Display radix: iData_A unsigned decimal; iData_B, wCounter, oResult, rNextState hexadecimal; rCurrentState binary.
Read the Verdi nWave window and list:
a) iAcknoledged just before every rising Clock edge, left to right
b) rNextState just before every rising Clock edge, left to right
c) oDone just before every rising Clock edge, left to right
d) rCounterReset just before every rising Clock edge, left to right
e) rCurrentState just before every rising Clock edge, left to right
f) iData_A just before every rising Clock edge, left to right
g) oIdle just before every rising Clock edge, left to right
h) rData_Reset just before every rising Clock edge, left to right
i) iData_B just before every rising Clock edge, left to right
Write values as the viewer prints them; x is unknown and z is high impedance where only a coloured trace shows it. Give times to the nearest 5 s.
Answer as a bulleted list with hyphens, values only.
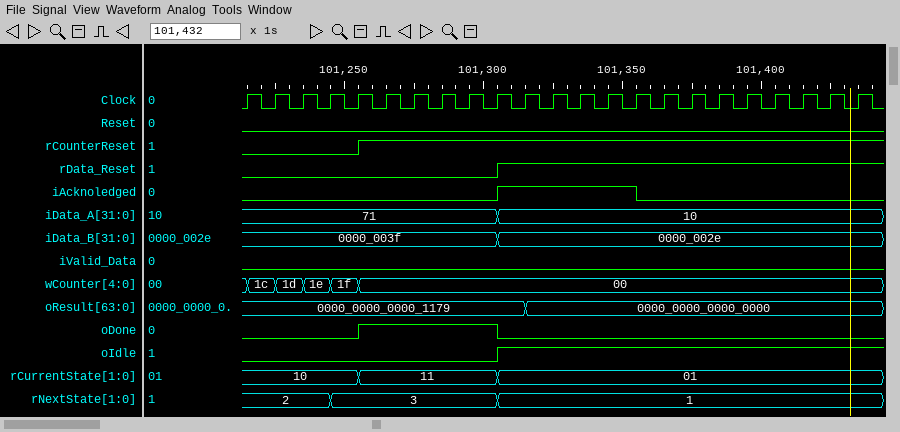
- 0 0 0 0 0 0 0 0 0 0 1 1 1 1 1 0 0 0 0 0 0 0 0
- 2, 2, 2, 2, 3, 3, 3, 3, 3, 3, 1, 1, 1, 1, 1, 1, 1, 1, 1, 1, 1, 1, 1
- 0 0 0 0 0 1 1 1 1 1 0 0 0 0 0 0 0 0 0 0 0 0 0
- 0 0 0 0 0 1 1 1 1 1 1 1 1 1 1 1 1 1 1 1 1 1 1
- 10, 10, 10, 10, 10, 11, 11, 11, 11, 11, 01, 01, 01, 01, 01, 01, 01, 01, 01, 01, 01, 01, 01
- 71, 71, 71, 71, 71, 71, 71, 71, 71, 71, 10, 10, 10, 10, 10, 10, 10, 10, 10, 10, 10, 10, 10
- 0 0 0 0 0 0 0 0 0 0 1 1 1 1 1 1 1 1 1 1 1 1 1
- 0 0 0 0 0 0 0 0 0 0 1 1 1 1 1 1 1 1 1 1 1 1 1
- 0000_003f, 0000_003f, 0000_003f, 0000_003f, 0000_003f, 0000_003f, 0000_003f, 0000_003f, 0000_003f, 0000_003f, 0000_002e, 0000_002e, 0000_002e, 0000_002e, 0000_002e, 0000_002e, 0000_002e, 0000_002e, 0000_002e, 0000_002e, 0000_002e, 0000_002e, 0000_002e
